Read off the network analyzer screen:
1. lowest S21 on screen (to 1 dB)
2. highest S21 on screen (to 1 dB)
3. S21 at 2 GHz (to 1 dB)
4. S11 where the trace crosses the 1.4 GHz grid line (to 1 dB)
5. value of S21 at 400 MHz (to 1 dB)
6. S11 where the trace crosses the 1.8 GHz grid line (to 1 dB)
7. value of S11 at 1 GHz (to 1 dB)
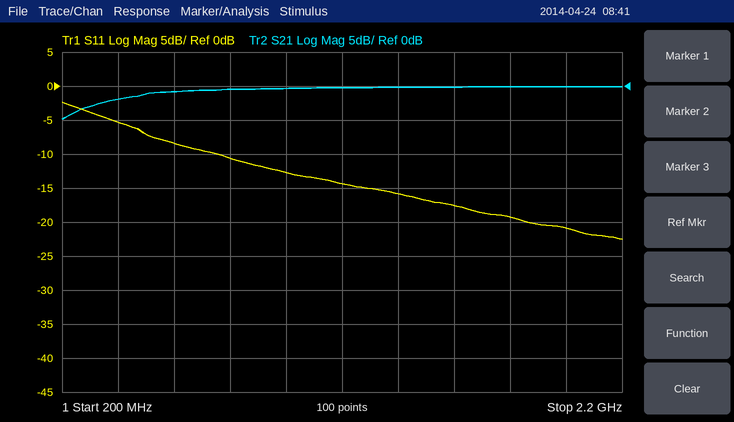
-5 dB
0 dB
0 dB
-16 dB
-2 dB
-19 dB
-13 dB
